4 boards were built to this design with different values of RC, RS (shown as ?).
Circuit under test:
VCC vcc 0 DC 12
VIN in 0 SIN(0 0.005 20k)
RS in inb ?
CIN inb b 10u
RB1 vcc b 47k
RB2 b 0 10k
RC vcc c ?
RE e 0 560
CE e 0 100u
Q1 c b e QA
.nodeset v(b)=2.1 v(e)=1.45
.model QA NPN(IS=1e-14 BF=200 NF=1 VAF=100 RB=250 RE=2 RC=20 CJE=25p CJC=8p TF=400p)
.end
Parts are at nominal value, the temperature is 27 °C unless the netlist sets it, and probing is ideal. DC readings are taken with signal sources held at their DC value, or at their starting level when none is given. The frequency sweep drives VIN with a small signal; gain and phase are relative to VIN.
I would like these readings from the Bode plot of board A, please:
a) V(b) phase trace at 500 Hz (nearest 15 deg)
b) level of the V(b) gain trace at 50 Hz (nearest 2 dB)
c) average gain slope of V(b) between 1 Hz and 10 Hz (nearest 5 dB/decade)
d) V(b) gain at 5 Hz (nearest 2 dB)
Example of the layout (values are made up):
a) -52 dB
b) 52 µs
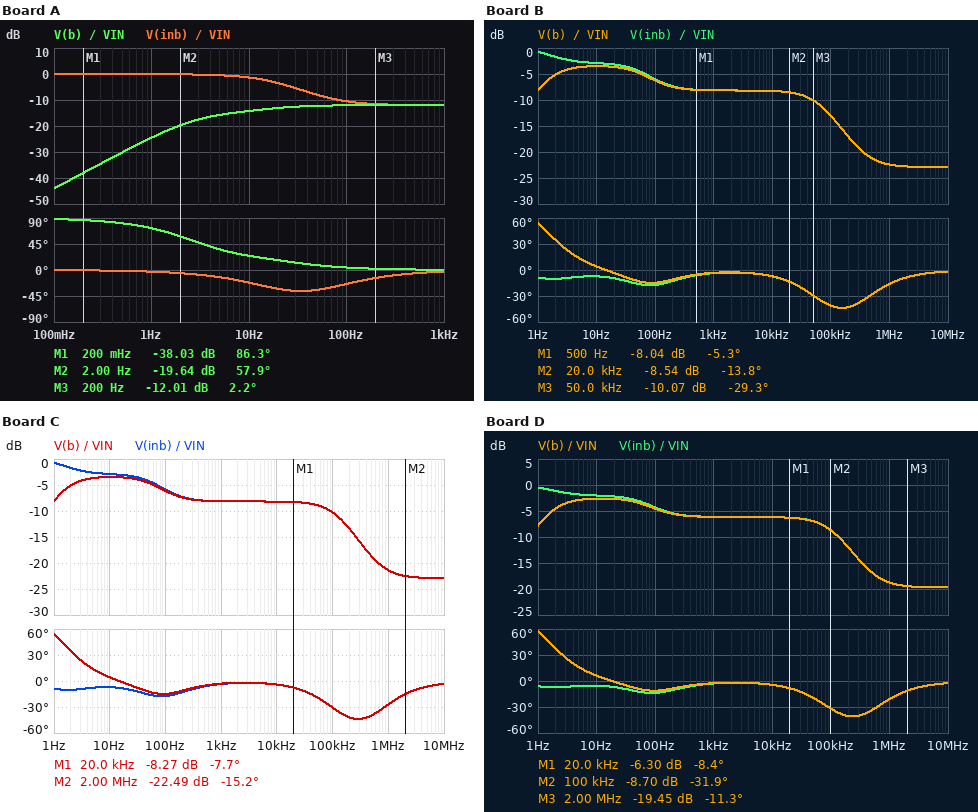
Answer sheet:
a) 0 deg
b) -12 dB
c) 10 dB/decade
d) -16 dB
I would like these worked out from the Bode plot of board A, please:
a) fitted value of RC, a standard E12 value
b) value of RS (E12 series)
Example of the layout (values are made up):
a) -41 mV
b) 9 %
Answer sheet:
a) 4.7 kΩ
b) 820 Ω
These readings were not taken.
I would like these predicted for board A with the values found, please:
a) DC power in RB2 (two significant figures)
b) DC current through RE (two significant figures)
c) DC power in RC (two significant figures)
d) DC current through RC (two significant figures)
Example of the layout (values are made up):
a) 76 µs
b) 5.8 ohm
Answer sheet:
a) 380 µW
b) 2.3 mA
c) 24 mW
d) 2.2 mA
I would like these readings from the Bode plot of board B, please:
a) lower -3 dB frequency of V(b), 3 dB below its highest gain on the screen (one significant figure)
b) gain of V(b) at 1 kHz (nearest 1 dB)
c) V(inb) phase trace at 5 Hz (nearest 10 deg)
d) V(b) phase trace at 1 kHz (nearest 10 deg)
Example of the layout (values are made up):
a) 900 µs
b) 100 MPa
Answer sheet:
a) 1 Hz
b) -8 dB
c) -10 deg
d) 0 deg
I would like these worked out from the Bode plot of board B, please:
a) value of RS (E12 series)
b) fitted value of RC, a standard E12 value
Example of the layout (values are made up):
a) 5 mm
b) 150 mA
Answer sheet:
a) 3.3 kΩ
b) 3.9 kΩ
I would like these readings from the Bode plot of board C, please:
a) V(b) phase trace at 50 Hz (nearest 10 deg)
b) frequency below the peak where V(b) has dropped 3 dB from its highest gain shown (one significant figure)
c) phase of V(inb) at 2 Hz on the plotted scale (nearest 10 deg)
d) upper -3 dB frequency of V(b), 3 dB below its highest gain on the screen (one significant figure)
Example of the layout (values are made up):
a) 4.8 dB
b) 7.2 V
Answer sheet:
a) -10 deg
b) 1 Hz
c) -10 deg
d) 100 Hz
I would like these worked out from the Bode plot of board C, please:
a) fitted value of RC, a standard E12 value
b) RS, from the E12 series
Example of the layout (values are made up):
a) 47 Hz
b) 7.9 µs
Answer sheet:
a) 2.7 kΩ
b) 3.3 kΩ
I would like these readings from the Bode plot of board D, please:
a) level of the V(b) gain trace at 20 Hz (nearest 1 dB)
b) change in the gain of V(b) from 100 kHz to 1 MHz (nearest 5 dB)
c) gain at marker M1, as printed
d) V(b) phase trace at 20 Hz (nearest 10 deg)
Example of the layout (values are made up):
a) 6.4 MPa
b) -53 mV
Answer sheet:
a) -3 dB
b) -10 dB
c) -6.30 dB
d) 0 deg
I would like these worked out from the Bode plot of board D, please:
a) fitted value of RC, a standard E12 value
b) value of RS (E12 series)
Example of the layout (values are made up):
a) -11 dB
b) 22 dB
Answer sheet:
a) 3.3 kΩ
b) 2.2 kΩ
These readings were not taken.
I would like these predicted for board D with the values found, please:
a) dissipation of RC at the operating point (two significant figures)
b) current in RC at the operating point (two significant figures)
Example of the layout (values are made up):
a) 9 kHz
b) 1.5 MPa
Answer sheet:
a) 18 mW
b) 2.4 mA
